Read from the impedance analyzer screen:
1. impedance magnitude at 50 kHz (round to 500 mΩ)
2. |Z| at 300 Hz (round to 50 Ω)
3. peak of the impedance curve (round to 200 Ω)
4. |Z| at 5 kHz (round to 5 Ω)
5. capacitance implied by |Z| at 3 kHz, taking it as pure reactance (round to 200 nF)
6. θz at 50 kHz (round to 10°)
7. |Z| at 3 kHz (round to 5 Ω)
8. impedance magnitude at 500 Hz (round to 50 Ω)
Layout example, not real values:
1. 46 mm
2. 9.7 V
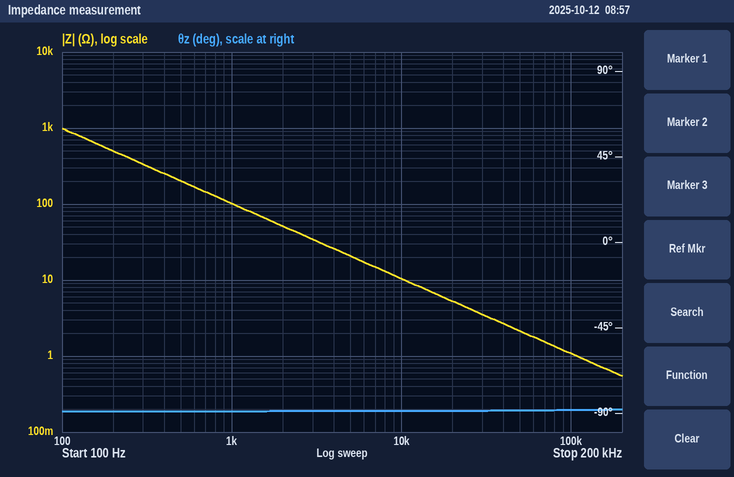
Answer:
1. 2.0 Ω
2. 350 Ω
3. 1.0 kΩ
4. 20 Ω
5. 1.6 µF
6. -90°
7. 35 Ω
8. 200 Ω
